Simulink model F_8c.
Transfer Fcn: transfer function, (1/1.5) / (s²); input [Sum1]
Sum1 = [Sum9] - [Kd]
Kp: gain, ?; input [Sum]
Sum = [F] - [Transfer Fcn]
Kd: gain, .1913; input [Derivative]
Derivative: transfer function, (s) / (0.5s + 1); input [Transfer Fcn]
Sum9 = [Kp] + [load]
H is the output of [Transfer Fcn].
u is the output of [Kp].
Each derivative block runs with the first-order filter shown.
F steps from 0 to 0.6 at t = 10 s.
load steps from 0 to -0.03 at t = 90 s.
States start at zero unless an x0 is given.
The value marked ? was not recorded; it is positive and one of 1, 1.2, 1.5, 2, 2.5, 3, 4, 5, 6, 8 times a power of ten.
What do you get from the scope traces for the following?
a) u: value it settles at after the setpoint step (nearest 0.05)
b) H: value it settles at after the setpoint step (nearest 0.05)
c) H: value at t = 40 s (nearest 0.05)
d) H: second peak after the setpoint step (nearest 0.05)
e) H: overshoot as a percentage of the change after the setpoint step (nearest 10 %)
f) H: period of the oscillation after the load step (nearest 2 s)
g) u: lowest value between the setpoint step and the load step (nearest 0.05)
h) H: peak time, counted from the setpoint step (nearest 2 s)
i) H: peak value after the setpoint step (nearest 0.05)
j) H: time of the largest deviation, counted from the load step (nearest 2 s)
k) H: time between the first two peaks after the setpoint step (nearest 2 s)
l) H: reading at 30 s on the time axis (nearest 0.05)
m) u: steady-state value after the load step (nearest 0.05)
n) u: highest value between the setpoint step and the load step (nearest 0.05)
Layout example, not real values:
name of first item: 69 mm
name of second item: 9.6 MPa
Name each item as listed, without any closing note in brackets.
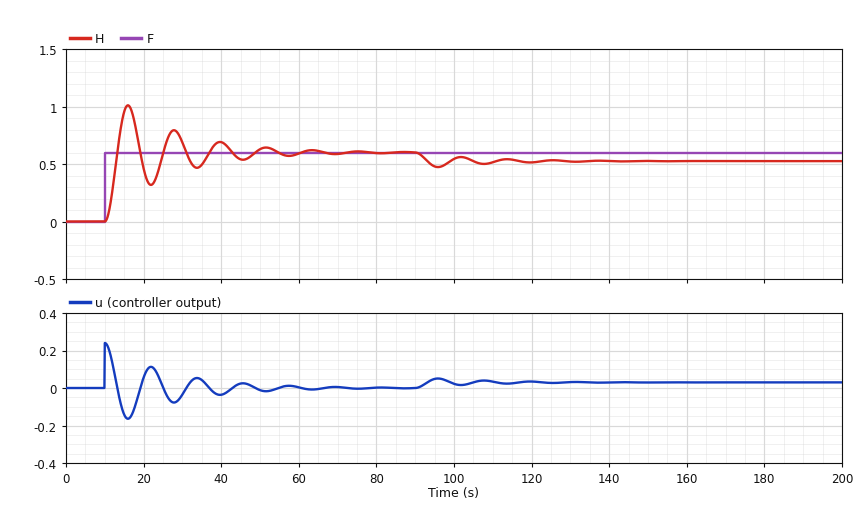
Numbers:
u: value it settles at after the setpoint step: 0.00
H: value it settles at after the setpoint step: 0.60
H: value at t = 40 s: 0.70
H: second peak after the setpoint step: 0.80
H: overshoot as a percentage of the change after the setpoint step: 70 %
H: period of the oscillation after the load step: 12 s
u: lowest value between the setpoint step and the load step: -0.15
H: peak time, counted from the setpoint step: 6 s
H: peak value after the setpoint step: 1.00
H: time of the largest deviation, counted from the load step: 6 s
H: time between the first two peaks after the setpoint step: 12 s
H: reading at 30 s on the time axis: 0.70
u: steady-state value after the load step: 0.05
u: highest value between the setpoint step and the load step: 0.25
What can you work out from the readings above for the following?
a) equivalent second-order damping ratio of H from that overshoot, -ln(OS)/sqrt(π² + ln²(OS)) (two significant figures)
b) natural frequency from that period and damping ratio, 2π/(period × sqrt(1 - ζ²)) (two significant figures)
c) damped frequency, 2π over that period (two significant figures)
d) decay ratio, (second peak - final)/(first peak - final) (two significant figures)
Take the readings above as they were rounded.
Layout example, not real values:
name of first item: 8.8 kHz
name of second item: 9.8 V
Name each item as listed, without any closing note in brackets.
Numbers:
equivalent second-order damping ratio of H from that overshoot, -ln(OS)/sqrt(π² + ln²(OS)): 0.11
natural frequency from that period and damping ratio, 2π/(period × sqrt(1 - ζ²)): 0.53 rad/s
damped frequency, 2π over that period: 0.52 rad/s
decay ratio, (second peak - final)/(first peak - final): 0.50
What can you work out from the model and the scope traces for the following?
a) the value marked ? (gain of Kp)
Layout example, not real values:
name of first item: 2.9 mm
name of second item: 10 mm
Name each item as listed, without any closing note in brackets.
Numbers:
the value marked ?: 0.4
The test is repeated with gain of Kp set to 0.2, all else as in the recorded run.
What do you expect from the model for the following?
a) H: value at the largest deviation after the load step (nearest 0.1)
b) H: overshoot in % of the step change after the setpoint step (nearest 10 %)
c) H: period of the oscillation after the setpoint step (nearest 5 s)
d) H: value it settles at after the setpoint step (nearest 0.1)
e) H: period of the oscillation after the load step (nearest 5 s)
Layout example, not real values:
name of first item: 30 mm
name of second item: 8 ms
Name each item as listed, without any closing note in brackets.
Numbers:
H: value at the largest deviation after the load step: 0.4
H: overshoot in % of the step change after the setpoint step: 60 %
H: period of the oscillation after the setpoint step: 15 s
H: value it settles at after the setpoint step: 0.6
H: period of the oscillation after the load step: 15 s
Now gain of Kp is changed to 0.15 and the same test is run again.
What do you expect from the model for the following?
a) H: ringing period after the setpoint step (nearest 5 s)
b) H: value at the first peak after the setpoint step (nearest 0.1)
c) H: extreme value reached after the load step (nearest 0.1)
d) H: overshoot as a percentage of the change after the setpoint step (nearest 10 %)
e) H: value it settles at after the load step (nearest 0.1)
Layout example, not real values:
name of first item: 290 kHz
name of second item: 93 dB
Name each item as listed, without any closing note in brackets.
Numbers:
H: ringing period after the setpoint step: 20 s
H: value at the first peak after the setpoint step: 0.9
H: extreme value reached after the load step: 0.3
H: overshoot as a percentage of the change after the setpoint step: 50 %
H: value it settles at after the load step: 0.4
